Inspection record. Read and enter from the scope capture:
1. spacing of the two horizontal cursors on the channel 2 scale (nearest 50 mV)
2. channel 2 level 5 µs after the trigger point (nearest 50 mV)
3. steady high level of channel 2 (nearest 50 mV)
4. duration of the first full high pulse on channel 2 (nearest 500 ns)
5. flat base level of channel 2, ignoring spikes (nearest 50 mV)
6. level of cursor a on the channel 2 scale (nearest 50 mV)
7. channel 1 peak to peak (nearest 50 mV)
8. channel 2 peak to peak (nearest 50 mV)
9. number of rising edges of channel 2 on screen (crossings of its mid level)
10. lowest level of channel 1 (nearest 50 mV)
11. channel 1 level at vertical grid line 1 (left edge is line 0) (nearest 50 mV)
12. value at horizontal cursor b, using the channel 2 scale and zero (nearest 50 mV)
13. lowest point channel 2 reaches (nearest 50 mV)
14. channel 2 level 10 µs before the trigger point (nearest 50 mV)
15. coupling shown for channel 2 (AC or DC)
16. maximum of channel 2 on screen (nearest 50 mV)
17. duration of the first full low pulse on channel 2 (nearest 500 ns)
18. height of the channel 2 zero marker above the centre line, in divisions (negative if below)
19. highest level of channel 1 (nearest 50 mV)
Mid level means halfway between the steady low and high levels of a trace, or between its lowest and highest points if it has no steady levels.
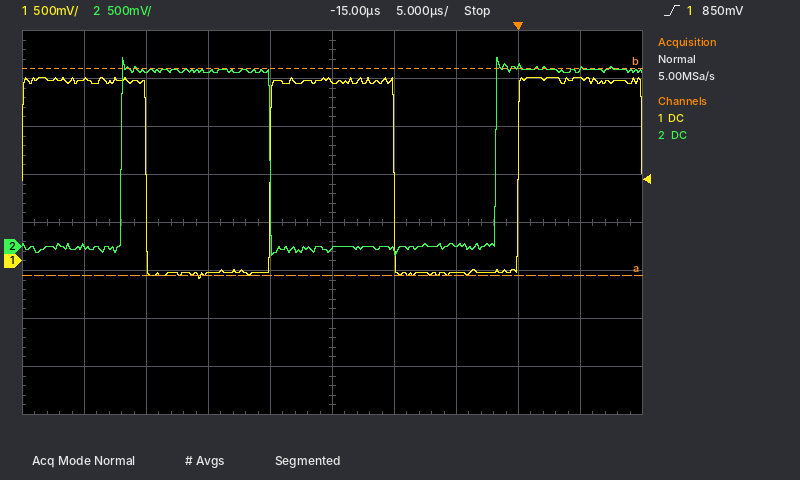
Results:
2.15 V
1.85 V
1.85 V
12.0 µs
0 mV
-300 mV
2.10 V
2.05 V
2
-200 mV
1.90 V
1.85 V
-100 mV
-50 mV
DC
1.95 V
18.0 µs
-0.5 div
1.90 V
